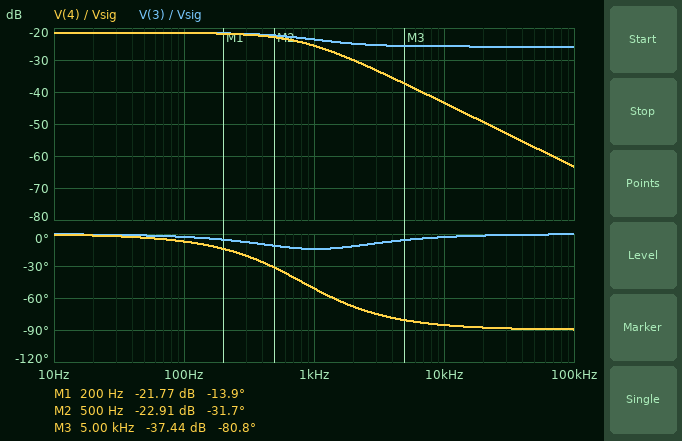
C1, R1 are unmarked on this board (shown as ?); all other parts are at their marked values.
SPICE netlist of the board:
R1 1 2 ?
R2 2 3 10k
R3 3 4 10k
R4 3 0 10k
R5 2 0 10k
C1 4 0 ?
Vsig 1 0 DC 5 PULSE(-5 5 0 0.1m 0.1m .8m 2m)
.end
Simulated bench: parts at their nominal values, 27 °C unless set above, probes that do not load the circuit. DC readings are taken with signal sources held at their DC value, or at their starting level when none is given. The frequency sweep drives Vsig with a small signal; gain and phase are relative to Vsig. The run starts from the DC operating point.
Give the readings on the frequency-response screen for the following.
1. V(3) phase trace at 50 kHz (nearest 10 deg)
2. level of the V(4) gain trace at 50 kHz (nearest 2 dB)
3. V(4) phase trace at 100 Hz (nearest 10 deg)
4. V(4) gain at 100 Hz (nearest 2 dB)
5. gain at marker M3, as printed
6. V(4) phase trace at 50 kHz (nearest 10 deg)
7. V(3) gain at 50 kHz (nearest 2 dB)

0 deg
-58 dB
-10 deg
-22 dB
-37.44 dB
-90 deg
-26 dB
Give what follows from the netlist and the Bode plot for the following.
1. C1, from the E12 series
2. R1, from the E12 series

12 nF
33 kΩ
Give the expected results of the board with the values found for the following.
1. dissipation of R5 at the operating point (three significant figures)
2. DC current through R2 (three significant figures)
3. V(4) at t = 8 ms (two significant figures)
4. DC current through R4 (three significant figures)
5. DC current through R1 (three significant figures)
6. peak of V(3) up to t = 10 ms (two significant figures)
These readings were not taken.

70.6 µW
42.0 µA
-420 mV
42.0 µA
126 µA
420 mV
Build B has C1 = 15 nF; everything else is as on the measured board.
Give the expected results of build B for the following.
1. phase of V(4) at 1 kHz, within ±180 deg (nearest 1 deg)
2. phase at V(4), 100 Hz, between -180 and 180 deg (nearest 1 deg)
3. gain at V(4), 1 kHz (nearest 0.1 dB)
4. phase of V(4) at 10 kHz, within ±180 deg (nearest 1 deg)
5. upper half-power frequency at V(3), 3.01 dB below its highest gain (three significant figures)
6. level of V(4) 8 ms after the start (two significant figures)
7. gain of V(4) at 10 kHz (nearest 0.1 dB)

-57 deg
-9 deg
-26.8 dB
-86 deg
1.28 kHz
-410 mV
-45.3 dB
